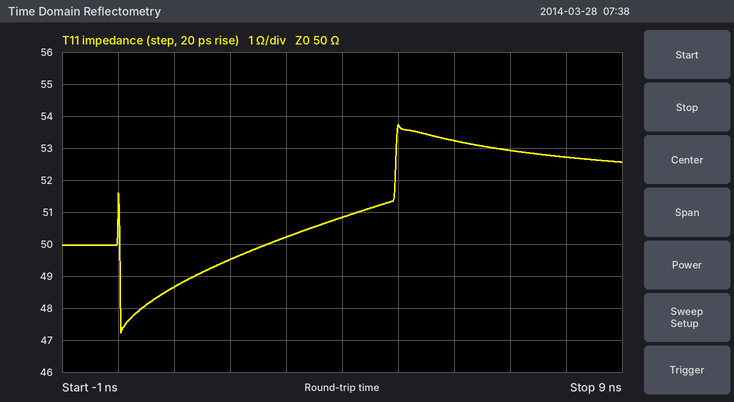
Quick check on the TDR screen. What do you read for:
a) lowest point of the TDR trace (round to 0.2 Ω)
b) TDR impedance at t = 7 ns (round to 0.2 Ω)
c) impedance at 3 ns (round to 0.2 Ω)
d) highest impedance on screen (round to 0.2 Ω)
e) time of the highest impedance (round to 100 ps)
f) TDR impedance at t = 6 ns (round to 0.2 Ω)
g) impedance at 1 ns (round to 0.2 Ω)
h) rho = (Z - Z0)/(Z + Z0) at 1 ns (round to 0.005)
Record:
47.2 Ω
53.0 Ω
50.2 Ω
53.8 Ω
5.0 ns
53.2 Ω
48.6 Ω
-0.015
